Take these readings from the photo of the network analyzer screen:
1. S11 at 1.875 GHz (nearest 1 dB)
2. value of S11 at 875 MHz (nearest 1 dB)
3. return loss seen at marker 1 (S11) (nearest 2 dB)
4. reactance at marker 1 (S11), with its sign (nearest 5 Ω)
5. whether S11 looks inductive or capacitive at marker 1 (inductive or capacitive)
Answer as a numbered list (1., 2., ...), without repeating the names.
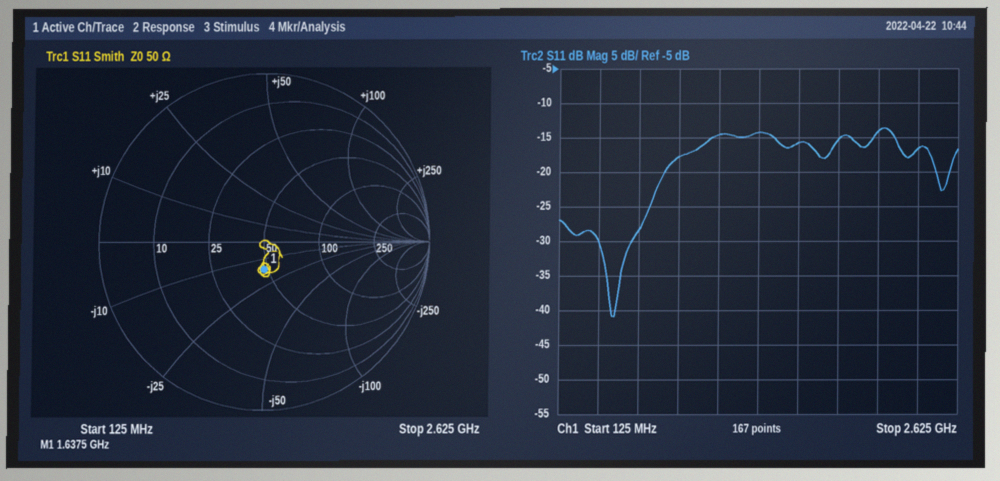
1. -15 dB
2. -18 dB
3. 16 dB
4. -15 Ω
5. capacitive
